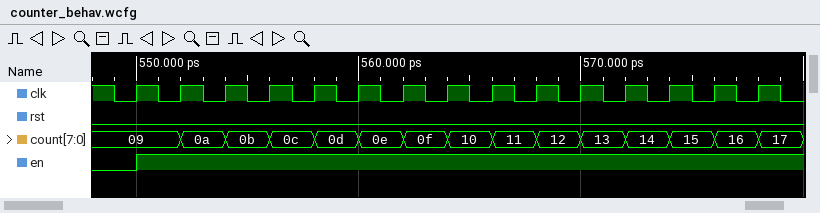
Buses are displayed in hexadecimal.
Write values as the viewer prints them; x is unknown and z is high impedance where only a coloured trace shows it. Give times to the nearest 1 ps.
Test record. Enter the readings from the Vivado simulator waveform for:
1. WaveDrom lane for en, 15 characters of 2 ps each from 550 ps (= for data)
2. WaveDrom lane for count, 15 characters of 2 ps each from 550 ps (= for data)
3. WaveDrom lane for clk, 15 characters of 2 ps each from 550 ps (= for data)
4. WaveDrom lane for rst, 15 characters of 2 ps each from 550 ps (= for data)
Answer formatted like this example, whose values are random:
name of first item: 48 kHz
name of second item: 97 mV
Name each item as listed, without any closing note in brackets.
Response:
WaveDrom lane for en, 15 characters of 2 ps each from 550 ps: {name: 'en', wave: '1..............'}
WaveDrom lane for count, 15 characters of 2 ps each from 550 ps: {name: 'count', wave: '===============', data: '09 0a 0b 0c 0d 0e 0f 10 11 12 13 14 15 16 17'}
WaveDrom lane for clk, 15 characters of 2 ps each from 550 ps: {name: 'clk', wave: 'p..............'}
WaveDrom lane for rst, 15 characters of 2 ps each from 550 ps: {name: 'rst', wave: '0..............'}
